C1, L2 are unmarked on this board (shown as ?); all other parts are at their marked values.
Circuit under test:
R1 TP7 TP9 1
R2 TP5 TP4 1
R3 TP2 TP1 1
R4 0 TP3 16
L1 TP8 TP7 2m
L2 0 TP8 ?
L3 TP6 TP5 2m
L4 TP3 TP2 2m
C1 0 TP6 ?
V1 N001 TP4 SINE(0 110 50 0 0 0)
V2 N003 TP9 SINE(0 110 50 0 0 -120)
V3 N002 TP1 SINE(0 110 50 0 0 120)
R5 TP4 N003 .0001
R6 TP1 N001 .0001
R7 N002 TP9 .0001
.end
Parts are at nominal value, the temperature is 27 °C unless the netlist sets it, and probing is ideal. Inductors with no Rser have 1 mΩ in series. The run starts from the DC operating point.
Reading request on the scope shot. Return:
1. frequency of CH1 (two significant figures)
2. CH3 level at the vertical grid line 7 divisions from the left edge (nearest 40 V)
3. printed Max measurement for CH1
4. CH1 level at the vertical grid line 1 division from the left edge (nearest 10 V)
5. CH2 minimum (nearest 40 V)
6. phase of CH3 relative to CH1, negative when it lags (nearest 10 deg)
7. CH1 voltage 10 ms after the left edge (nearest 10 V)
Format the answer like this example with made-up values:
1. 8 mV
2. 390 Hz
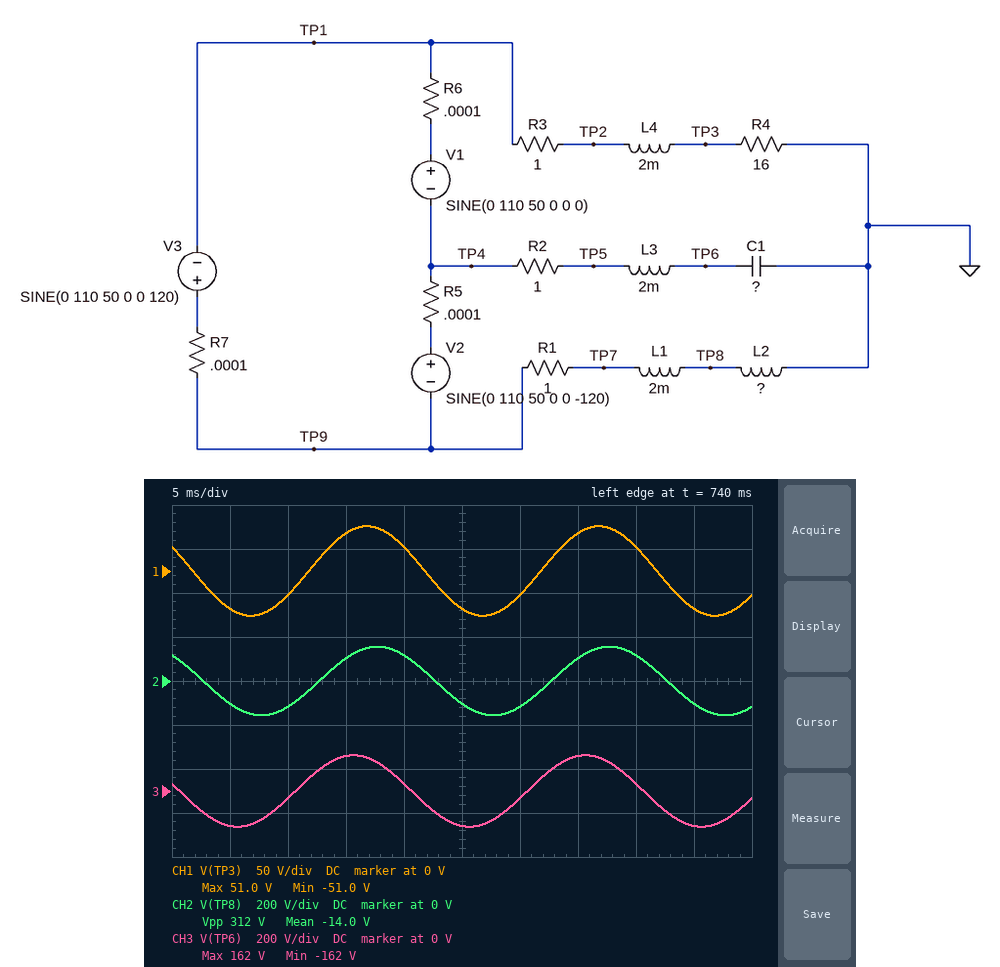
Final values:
1. 50 Hz
2. 160 V
3. 51.0 V
4. -40 V
5. -160 V
6. 20 deg
7. -30 V
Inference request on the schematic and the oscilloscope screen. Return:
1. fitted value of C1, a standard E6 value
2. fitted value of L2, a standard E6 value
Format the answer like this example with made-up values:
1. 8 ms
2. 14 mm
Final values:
1. 100 µF
2. 100 mH
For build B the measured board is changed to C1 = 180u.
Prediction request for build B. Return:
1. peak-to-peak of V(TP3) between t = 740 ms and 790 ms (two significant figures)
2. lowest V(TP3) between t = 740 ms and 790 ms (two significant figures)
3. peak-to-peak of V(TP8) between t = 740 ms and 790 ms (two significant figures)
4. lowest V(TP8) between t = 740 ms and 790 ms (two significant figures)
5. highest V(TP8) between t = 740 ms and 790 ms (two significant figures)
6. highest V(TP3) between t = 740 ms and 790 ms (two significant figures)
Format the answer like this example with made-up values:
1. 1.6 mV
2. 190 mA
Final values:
1. 150 V
2. -73 V
3. 360 V
4. -180 V
5. 180 V
6. 73 V
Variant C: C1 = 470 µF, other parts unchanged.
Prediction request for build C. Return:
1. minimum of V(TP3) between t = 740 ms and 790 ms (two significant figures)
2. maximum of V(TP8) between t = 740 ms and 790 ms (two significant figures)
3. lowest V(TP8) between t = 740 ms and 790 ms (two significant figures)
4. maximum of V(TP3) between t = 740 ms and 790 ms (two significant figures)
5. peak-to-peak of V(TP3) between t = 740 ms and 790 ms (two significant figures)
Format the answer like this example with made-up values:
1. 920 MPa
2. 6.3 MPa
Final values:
1. -97 V
2. 150 V
3. -150 V
4. 97 V
5. 190 V
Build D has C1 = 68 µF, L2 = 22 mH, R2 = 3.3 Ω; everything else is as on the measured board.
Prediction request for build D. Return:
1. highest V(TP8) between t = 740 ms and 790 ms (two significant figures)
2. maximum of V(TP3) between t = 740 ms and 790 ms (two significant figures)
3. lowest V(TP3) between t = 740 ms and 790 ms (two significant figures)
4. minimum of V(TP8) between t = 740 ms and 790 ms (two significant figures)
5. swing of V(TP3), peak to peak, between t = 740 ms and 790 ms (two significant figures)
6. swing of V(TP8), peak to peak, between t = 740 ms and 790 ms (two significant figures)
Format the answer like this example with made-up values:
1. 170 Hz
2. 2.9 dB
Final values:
1. 58 V
2. 90 V
3. -90 V
4. -58 V
5. 180 V
6. 120 V
